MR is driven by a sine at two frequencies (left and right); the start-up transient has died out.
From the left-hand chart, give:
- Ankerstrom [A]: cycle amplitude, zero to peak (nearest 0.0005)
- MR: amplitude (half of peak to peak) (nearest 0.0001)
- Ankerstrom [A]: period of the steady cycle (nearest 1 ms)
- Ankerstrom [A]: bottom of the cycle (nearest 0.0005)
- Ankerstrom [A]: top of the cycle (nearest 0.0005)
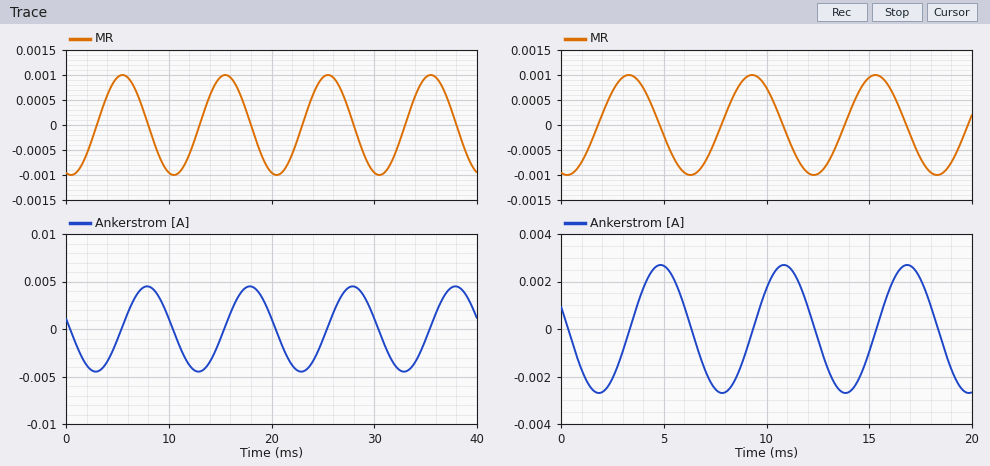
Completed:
0.0045
0.0010
10 ms
-0.0045
0.0045
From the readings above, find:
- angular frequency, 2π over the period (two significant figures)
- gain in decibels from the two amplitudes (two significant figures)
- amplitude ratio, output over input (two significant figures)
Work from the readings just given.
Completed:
0.63 rad/ms
13 dB
4.5
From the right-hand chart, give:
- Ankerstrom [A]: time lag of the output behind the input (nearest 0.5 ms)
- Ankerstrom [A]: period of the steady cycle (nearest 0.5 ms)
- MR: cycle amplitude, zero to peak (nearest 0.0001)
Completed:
1.5 ms
6.0 ms
0.0010
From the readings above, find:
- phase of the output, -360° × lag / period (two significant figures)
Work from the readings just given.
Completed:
-90°
